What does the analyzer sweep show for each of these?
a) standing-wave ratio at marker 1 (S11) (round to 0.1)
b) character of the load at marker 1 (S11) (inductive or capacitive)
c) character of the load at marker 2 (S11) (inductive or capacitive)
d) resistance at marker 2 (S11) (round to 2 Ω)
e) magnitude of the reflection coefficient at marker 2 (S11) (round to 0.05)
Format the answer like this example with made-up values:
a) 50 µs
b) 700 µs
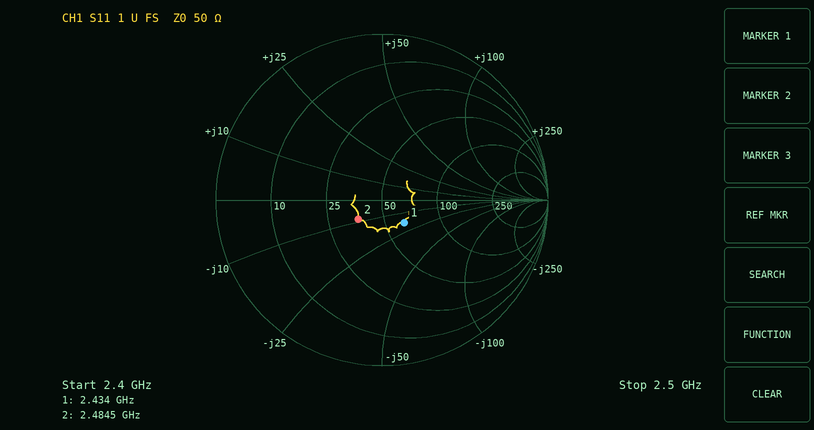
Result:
a) 1.5
b) capacitive
c) capacitive
d) 36 Ω
e) 0.20
